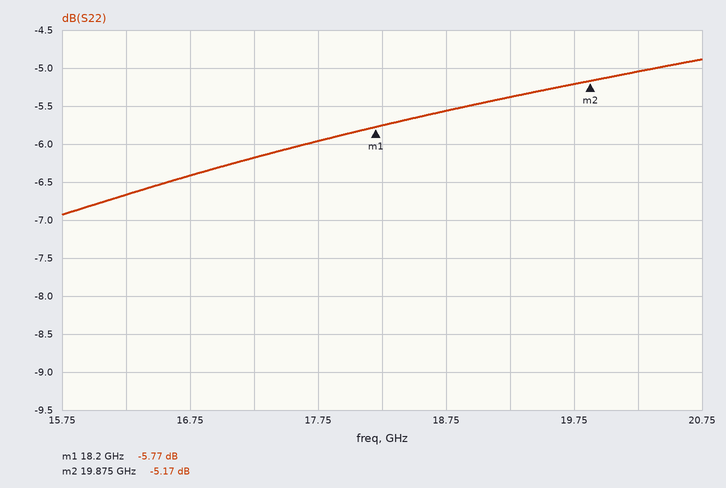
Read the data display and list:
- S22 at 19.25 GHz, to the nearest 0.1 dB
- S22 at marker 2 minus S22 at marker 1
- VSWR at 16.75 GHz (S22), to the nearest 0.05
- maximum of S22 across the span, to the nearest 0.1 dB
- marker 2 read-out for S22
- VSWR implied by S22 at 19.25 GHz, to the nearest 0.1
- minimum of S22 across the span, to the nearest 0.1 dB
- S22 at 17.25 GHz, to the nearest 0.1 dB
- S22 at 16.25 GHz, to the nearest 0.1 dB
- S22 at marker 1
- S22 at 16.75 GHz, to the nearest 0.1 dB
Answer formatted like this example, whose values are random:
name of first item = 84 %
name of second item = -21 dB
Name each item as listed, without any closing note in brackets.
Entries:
S22 at 19.25 GHz, to the nearest 0.1 dB = -5.4 dB
S22 at marker 2 minus S22 at marker 1 = 0.60 dB
VSWR at 16.75 GHz (S22), to the nearest 0.05 = 2.85
maximum of S22 across the span, to the nearest 0.1 dB = -4.9 dB
marker 2 read-out for S22 = -5.17 dB
VSWR implied by S22 at 19.25 GHz, to the nearest 0.1 = 3.3
minimum of S22 across the span, to the nearest 0.1 dB = -6.9 dB
S22 at 17.25 GHz, to the nearest 0.1 dB = -6.2 dB
S22 at 16.25 GHz, to the nearest 0.1 dB = -6.7 dB
S22 at marker 1 = -5.77 dB
S22 at 16.75 GHz, to the nearest 0.1 dB = -6.4 dB
